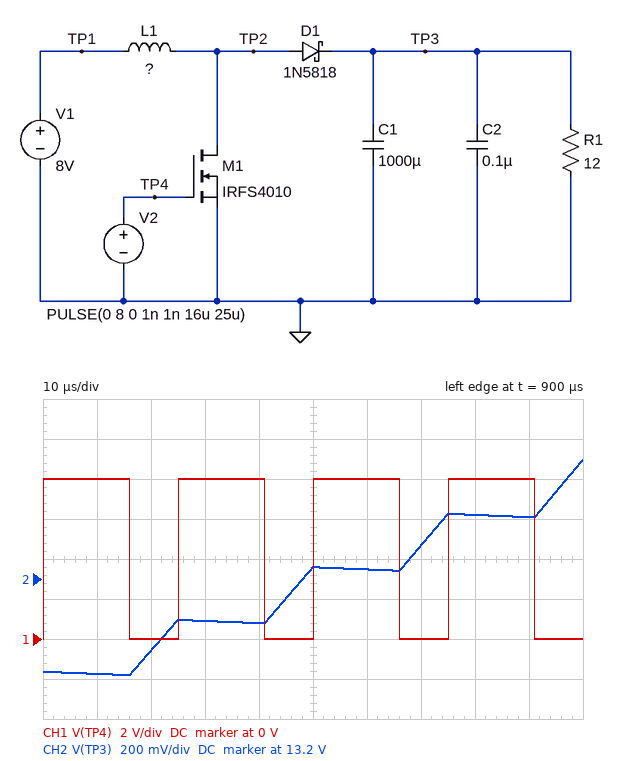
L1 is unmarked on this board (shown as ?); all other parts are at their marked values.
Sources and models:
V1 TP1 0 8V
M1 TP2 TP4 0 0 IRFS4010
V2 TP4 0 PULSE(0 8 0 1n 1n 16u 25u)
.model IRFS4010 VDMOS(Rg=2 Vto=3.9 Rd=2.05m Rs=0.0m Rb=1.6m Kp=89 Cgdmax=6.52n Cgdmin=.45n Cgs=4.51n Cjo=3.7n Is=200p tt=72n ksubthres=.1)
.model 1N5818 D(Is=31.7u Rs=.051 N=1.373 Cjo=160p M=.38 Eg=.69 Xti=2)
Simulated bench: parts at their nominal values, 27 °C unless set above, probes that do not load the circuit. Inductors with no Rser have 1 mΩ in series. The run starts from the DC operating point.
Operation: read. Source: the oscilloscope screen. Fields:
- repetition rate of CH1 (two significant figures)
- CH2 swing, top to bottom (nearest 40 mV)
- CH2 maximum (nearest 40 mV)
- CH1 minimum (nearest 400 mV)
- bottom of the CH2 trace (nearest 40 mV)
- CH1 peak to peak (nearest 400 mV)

40 kHz
1.08 V
13.80 V
0 V
12.72 V
8.0 V
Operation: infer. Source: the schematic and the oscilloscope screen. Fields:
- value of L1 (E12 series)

120 µH
